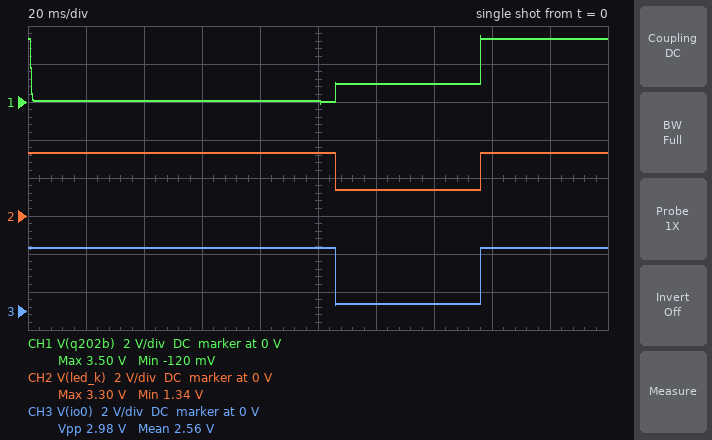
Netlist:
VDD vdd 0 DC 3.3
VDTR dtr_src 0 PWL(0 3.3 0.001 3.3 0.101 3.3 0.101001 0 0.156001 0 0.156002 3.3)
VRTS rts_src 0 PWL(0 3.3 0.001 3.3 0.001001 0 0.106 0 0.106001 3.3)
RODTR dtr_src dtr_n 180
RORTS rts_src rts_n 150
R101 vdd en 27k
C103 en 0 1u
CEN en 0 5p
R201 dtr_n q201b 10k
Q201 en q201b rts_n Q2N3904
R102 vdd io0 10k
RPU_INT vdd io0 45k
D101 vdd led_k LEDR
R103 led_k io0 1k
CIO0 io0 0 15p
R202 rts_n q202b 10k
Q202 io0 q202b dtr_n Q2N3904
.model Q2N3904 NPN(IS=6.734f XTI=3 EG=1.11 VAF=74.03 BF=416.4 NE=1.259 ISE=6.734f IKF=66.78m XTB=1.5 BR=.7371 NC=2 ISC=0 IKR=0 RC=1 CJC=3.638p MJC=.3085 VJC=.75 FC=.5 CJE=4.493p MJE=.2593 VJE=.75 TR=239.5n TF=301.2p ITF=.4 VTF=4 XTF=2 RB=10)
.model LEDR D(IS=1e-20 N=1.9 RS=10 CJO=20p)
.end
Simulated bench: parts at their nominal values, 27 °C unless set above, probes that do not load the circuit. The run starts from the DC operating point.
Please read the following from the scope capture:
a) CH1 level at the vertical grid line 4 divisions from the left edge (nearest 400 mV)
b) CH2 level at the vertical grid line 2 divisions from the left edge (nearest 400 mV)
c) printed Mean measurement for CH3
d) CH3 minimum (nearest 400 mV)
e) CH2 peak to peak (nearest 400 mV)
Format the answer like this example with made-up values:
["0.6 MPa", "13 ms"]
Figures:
["0 V", "3.2 V", "2.56 V", "400 mV", "2.0 V"]
